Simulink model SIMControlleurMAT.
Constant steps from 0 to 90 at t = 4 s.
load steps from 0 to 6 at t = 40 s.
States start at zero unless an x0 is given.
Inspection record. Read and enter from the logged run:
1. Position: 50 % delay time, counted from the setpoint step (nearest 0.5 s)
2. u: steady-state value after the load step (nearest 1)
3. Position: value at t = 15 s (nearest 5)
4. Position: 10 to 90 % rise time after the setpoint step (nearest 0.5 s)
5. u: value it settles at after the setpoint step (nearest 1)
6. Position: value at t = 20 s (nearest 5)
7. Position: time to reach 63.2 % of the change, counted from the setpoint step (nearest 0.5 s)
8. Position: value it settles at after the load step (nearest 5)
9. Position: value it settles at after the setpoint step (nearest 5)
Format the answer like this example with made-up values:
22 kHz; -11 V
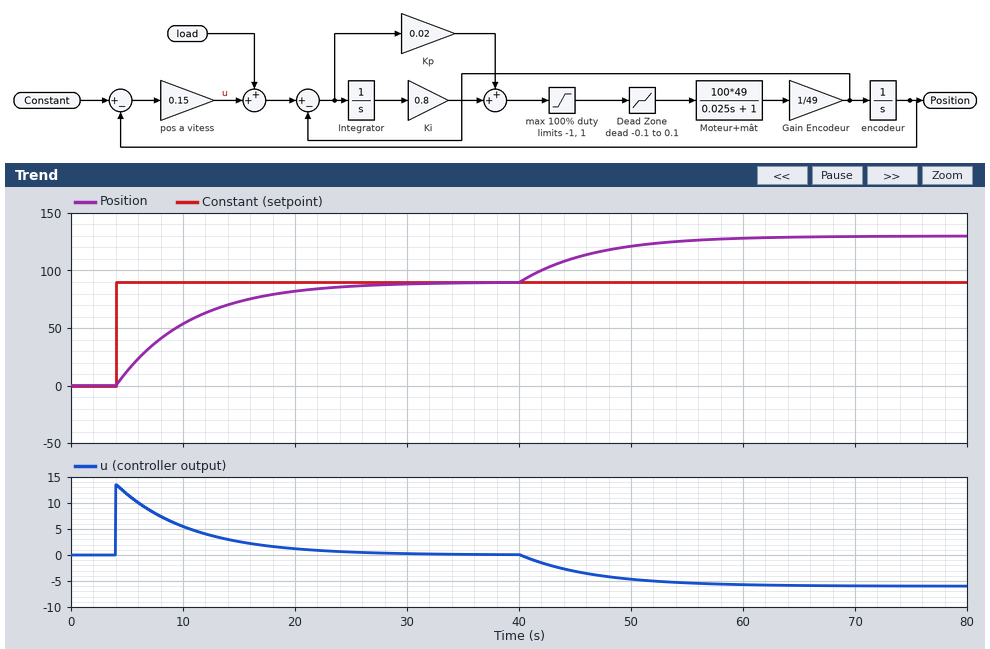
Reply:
4.5 s; -6; 75; 14.5 s; 0; 80; 6.5 s; 130; 90
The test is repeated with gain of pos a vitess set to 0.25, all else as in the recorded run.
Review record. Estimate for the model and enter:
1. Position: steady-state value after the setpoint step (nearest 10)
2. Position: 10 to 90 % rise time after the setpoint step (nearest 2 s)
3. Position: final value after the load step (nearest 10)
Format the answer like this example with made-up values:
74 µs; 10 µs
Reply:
90; 8 s; 110
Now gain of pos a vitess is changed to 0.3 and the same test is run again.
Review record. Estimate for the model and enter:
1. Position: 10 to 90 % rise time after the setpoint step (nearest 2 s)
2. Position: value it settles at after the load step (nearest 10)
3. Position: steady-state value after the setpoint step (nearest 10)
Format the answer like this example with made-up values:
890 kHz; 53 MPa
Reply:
8 s; 110; 90
